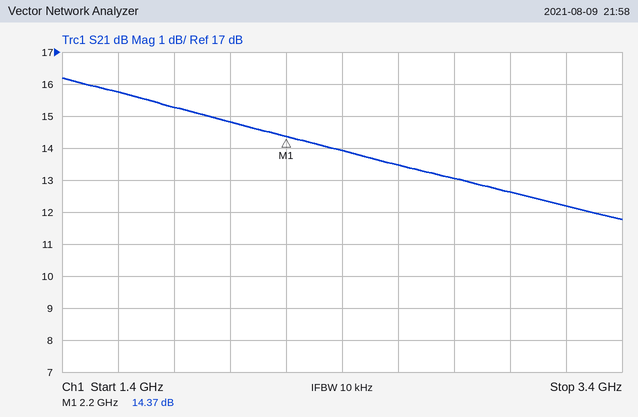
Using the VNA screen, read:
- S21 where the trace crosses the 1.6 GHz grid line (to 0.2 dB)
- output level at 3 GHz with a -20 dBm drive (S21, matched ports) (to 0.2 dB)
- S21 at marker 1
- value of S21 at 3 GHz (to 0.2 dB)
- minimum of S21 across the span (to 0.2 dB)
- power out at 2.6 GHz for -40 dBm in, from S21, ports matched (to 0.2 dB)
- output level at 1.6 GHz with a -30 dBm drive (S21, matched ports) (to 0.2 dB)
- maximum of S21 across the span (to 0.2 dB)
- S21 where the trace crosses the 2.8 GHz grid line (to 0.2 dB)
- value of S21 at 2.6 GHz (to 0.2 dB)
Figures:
15.8 dB
-7.4 dBm
14.37 dB
12.6 dB
11.8 dB
-26.6 dBm
-14.2 dBm
16.2 dB
13.0 dB
13.4 dB
